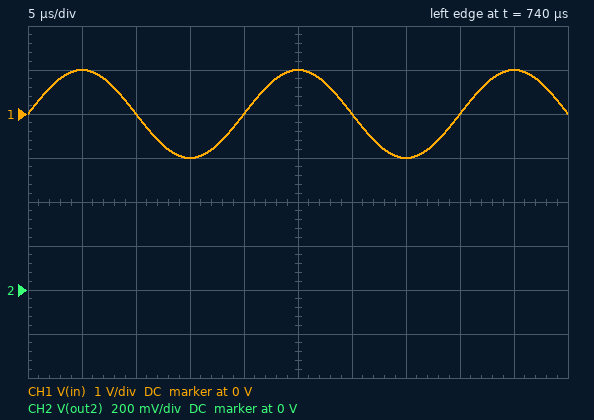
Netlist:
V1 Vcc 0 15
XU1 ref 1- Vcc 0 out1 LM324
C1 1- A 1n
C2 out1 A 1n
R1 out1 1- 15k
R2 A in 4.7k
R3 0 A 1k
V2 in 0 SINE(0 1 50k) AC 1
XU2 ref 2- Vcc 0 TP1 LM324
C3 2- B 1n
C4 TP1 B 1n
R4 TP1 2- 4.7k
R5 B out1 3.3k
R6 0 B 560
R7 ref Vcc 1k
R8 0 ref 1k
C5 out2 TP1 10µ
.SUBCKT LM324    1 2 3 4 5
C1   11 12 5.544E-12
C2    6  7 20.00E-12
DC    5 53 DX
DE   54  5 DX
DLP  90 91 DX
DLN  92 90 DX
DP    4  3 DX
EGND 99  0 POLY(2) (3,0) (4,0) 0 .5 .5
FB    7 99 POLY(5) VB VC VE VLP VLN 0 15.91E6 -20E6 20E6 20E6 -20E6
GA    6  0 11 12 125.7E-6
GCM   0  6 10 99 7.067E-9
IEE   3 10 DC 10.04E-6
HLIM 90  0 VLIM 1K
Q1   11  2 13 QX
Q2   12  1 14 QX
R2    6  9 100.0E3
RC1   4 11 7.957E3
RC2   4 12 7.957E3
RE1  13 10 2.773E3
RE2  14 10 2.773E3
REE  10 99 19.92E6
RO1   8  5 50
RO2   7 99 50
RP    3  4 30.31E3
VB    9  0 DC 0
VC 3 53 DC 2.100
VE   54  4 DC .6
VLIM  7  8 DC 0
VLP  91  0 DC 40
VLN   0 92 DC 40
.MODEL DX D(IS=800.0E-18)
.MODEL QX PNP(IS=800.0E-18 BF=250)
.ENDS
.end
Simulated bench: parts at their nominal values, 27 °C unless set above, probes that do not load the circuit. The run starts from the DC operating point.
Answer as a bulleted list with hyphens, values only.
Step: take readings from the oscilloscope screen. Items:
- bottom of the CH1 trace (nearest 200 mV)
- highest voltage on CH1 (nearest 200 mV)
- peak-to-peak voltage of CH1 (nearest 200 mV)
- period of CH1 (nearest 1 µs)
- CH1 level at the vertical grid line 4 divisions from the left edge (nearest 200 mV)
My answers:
- -1.0 V
- 1.0 V
- 2.0 V
- 20 µs
- 0 V
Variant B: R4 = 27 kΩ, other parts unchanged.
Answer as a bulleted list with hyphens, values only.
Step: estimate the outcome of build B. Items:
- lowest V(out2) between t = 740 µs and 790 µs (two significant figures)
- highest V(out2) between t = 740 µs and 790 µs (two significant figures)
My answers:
- 5.9 V
- 9.1 V
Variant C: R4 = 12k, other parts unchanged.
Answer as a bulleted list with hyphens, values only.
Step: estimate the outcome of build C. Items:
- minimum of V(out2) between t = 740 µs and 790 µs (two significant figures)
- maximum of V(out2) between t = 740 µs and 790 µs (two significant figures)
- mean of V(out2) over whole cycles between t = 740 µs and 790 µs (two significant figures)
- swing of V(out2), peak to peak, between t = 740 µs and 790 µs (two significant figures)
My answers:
- 5.6 V
- 9.4 V
- 7.5 V
- 3.8 V
